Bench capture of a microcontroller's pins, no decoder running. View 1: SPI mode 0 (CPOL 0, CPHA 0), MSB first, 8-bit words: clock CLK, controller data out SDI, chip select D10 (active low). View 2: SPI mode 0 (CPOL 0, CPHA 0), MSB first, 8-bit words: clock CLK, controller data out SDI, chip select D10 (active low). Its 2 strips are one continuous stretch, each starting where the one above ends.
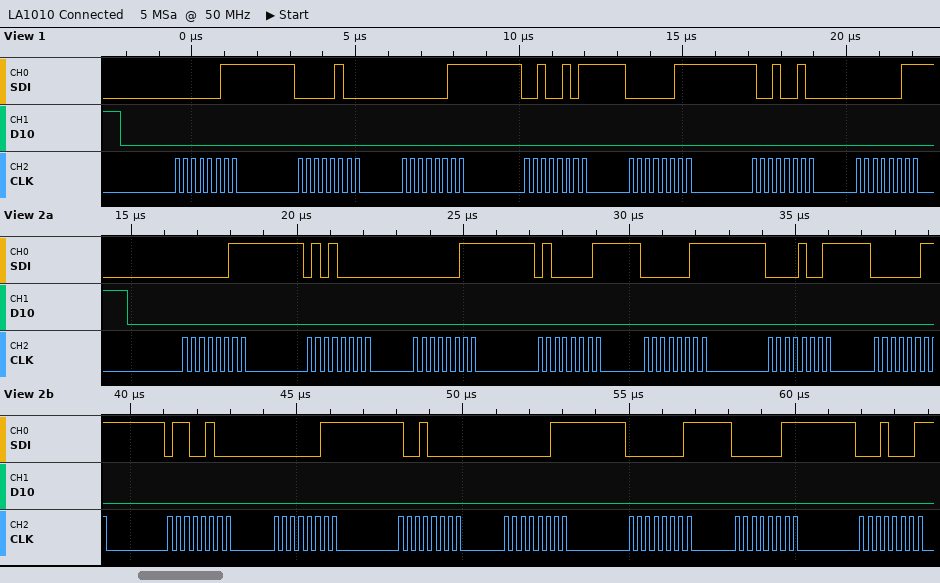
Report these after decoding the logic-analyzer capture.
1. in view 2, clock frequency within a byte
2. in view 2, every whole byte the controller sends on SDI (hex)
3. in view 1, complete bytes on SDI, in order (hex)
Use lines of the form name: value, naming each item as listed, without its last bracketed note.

in view 2, clock frequency within a byte: 4 MHz
in view 2, every whole byte the controller sends on SDI: 03 50 03 41 03 09 03 64 03 90 03 01 03 11
in view 1, complete bytes on SDI, in order: 03 04 03 25 03 92 03
